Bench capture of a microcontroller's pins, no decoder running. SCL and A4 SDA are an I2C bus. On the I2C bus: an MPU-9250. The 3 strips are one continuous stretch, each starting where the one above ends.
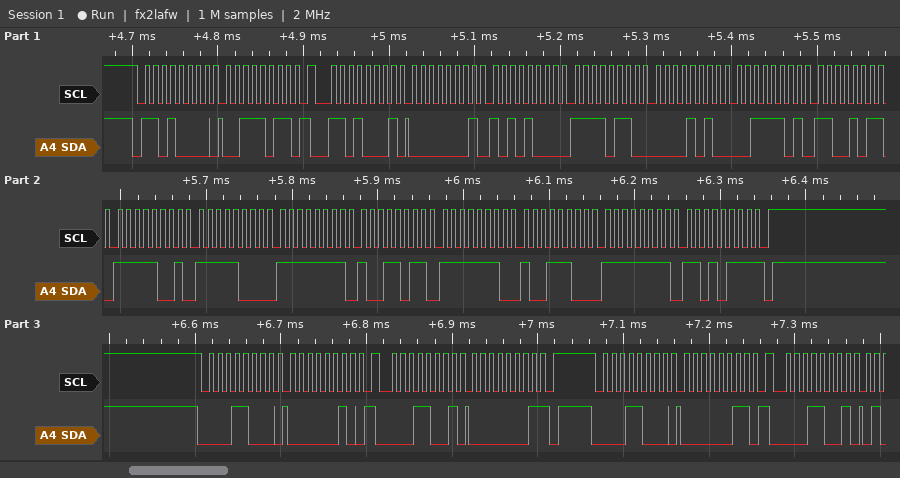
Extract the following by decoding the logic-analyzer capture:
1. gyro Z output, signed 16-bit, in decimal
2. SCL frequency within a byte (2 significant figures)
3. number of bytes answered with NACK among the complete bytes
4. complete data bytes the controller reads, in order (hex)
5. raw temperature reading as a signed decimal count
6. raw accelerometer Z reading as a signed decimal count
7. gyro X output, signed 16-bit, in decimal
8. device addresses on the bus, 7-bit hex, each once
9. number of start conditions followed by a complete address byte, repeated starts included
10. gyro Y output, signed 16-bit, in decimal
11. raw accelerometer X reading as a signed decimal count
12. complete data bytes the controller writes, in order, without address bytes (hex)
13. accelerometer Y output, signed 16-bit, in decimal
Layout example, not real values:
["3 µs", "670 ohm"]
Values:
["-41", "100 kHz", "2", "01 A8 F6 0A 3D CB F9 F8 FF 9B FE 9C FF D7 01", "-1544", "15819", "-101", "0x68 0x0C", "6", "-356", "424", "3B 02 03", "-2550"]
